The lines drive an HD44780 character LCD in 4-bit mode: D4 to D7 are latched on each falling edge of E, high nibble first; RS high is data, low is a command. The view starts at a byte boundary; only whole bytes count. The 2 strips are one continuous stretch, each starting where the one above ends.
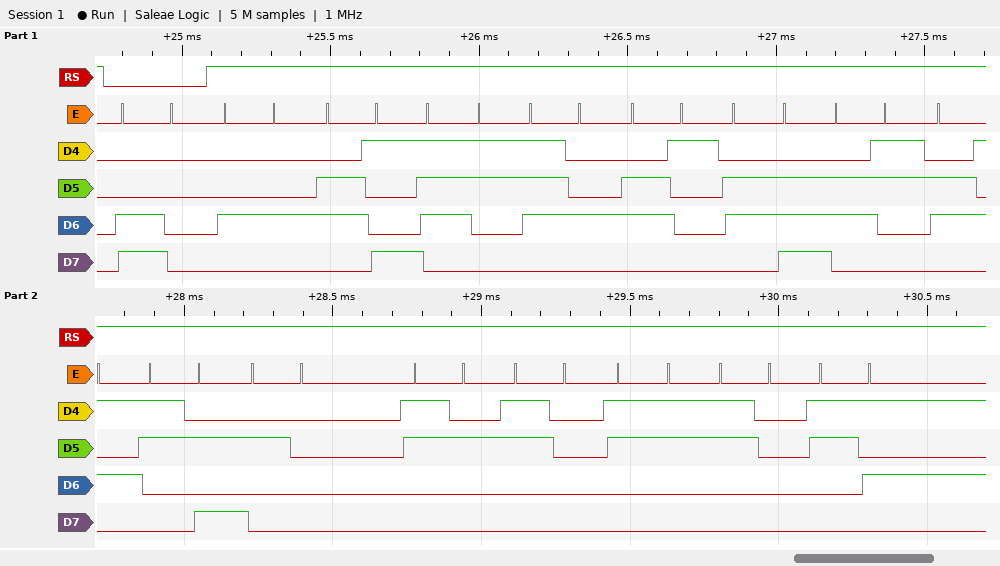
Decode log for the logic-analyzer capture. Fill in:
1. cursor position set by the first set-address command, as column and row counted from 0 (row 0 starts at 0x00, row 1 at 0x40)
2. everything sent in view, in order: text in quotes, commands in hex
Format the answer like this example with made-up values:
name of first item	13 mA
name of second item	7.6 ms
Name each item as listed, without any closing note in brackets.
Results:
cursor position set by the first set-address command, as column and row counted from 0	column 0, row 1
everything sent in view, in order: text in quotes, commands in hex	0xC0 "Distance: 20305"
